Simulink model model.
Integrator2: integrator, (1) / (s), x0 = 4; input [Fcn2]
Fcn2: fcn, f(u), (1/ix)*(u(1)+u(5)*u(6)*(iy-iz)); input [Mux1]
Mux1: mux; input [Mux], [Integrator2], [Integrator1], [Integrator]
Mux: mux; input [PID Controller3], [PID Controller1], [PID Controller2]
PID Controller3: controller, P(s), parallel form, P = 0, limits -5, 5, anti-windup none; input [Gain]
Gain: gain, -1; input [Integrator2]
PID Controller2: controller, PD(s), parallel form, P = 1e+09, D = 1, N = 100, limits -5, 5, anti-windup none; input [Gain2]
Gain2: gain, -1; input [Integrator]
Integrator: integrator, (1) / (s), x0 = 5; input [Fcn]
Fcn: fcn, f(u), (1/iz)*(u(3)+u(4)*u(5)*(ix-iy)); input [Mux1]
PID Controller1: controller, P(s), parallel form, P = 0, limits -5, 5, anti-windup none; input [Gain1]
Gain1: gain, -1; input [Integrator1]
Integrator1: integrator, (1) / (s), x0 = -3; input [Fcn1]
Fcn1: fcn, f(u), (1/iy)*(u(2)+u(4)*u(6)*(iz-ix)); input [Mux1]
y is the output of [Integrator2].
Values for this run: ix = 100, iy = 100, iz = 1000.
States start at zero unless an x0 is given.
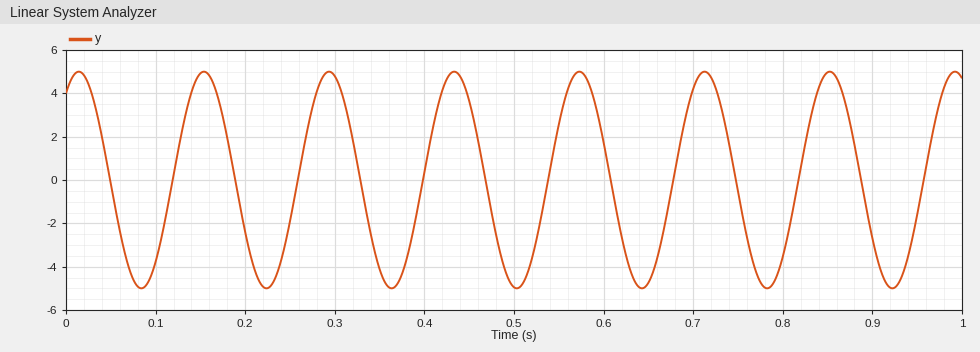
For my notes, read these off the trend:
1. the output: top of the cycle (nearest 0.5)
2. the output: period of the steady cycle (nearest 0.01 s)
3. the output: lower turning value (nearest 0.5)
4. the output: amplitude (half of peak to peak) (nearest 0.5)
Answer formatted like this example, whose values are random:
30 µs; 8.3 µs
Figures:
5.0; 0.14 s; -5.0; 5.0
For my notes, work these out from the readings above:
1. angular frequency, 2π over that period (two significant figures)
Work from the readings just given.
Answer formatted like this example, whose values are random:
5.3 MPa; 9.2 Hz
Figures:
45 rad/s
